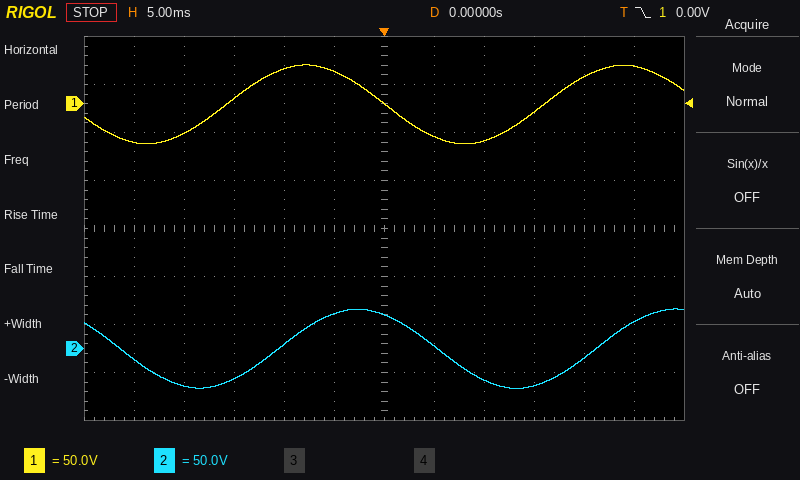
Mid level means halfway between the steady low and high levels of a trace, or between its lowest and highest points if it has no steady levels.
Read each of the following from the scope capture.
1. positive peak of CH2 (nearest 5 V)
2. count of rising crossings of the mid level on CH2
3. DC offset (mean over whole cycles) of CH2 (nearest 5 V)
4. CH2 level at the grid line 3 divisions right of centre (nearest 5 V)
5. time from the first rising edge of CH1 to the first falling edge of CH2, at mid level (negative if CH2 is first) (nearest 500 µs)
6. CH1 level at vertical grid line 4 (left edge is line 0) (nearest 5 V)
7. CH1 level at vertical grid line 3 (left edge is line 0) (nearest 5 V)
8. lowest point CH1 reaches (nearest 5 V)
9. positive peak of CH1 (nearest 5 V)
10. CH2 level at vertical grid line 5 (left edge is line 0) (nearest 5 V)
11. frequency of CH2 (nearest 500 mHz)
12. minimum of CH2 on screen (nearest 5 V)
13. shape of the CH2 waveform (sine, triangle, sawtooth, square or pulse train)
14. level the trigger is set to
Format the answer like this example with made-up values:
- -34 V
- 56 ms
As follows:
- 40 V
- 2
- 0 V
- -40 V
- -10.5 ms
- 35 V
- 5 V
- -40 V
- 40 V
- 35 V
- 31.5 Hz
- -40 V
- sine
- 0.00 V
